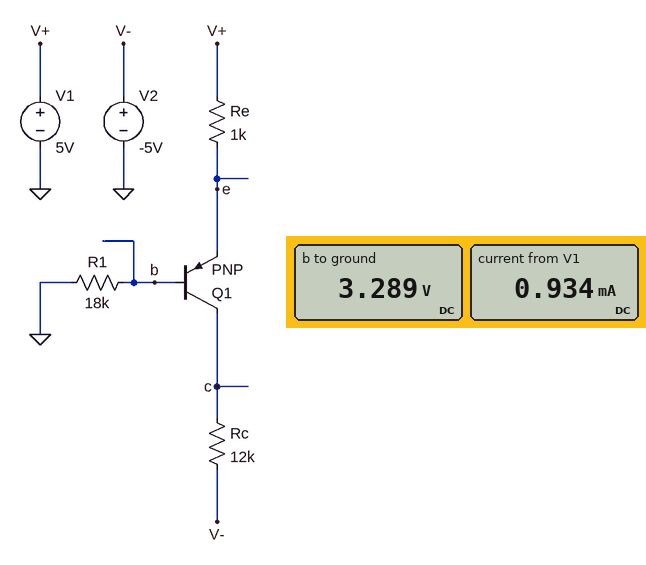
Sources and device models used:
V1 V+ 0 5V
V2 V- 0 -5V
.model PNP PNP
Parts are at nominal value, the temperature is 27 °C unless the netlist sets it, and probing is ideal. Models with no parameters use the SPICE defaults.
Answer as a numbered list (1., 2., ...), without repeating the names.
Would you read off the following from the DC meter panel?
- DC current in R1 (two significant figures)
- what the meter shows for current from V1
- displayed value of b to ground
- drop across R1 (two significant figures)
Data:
1. 180 µA
2. 0.934 mA
3. 3.289 V
4. 3.3 V
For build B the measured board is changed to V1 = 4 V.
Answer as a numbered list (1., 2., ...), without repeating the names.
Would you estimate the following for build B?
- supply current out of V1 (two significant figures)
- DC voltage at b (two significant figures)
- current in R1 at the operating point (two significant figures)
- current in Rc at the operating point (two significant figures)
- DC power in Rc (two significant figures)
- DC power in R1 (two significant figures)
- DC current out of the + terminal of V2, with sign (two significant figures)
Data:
1. 810 µA
2. 2.4 V
3. 130 µA
4. 680 µA
5. 5.5 mW
6. 320 µW
7. -680 µA
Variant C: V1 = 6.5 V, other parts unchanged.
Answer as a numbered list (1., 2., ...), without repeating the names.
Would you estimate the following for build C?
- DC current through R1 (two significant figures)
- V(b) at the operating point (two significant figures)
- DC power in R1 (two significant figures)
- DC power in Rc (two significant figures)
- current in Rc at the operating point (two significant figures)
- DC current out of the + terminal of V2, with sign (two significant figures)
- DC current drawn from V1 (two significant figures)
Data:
1. 260 µA
2. 4.6 V
3. 1.2 mW
4. 8.9 mW
5. 860 µA
6. -860 µA
7. 1.1 mA
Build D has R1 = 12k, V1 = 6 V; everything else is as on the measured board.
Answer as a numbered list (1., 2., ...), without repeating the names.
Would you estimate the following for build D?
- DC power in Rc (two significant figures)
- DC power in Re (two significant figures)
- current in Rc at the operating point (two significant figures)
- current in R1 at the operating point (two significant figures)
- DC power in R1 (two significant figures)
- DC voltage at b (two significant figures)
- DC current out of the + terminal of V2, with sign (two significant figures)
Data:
1. 8.0 mW
2. 1.3 mW
3. 820 µA
4. 340 µA
5. 1.4 mW
6. 4.1 V
7. -820 µA
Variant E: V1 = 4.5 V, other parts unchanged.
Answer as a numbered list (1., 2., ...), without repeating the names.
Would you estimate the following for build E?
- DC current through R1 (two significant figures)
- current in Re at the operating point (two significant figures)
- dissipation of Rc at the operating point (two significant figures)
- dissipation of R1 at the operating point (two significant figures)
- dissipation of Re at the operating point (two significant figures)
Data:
1. 160 µA
2. 870 µA
3. 6.1 mW
4. 450 µW
5. 760 µW
